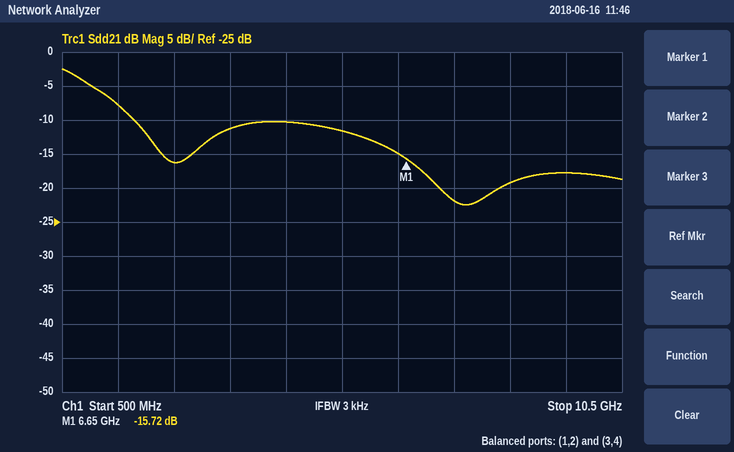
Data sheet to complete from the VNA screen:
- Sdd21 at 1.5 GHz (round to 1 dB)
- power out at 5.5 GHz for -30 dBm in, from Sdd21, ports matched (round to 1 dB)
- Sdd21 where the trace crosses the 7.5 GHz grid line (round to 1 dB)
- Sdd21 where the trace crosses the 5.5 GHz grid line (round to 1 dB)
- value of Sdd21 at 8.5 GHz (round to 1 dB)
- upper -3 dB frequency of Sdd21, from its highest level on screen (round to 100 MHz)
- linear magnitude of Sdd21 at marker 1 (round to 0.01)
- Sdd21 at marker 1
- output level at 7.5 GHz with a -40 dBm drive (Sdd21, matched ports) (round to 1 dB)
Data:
-8 dB
-42 dBm
-22 dB
-12 dB
-19 dB
1.1 GHz
0.16
-15.72 dB
-62 dBm
